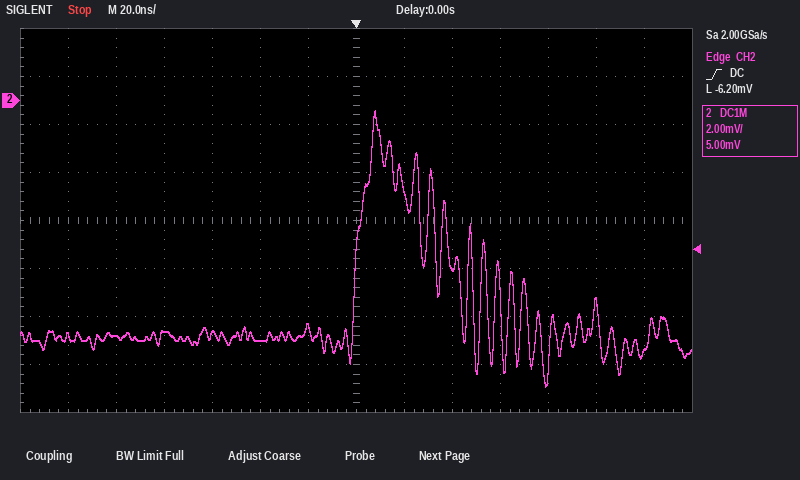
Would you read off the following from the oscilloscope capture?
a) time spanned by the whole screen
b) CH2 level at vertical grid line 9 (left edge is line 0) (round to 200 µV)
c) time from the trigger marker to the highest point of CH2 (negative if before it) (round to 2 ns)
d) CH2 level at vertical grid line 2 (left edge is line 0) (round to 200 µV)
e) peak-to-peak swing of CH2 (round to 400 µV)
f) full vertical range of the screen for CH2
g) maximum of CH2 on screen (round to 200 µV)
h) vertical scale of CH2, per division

280 ns
-7.0 mV
+8 ns
-9.8 mV
11.6 mV
16 mV
-400 µV
2 mV
